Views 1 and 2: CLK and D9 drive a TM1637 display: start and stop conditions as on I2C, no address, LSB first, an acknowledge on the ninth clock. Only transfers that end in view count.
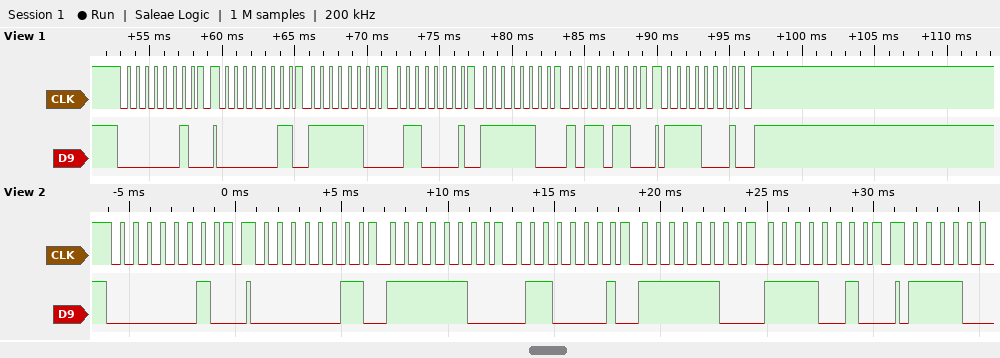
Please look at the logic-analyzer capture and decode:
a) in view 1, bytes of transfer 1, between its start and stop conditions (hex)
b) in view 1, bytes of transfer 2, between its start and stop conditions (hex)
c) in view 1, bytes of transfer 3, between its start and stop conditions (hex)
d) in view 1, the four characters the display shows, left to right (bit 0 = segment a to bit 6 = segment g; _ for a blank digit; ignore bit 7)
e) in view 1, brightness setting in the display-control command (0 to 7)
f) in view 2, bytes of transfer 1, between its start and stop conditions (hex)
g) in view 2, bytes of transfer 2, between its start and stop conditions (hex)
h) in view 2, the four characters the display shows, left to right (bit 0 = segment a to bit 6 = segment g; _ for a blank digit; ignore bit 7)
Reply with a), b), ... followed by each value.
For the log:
a) 40
b) C0 3F 86 3F 6D
c) 8F
d) 0105
e) 7
f) 40
g) C0 3F 86 3F 4F
h) 0103
